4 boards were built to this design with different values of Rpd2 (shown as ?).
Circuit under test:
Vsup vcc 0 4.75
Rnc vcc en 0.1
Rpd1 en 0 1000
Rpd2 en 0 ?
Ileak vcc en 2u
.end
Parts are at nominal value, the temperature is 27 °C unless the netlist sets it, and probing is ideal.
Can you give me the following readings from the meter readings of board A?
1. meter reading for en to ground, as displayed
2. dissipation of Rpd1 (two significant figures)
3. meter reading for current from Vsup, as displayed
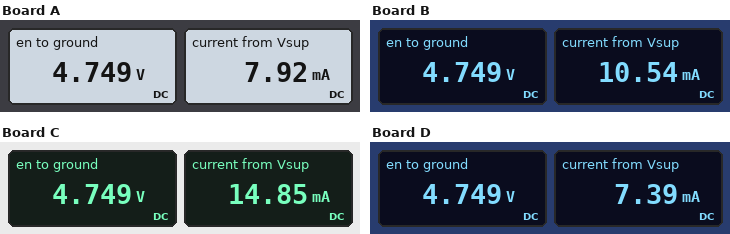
4.749 V
23 mW
7.92 mA
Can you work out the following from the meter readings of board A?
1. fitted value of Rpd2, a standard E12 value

1.5 kΩ
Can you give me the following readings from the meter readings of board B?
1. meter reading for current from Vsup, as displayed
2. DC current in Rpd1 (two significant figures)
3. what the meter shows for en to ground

10.54 mA
4.7 mA
4.749 V
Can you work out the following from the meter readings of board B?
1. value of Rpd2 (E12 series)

820 Ω
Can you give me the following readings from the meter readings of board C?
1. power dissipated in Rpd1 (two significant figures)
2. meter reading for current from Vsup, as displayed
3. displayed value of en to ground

23 mW
14.85 mA
4.749 V
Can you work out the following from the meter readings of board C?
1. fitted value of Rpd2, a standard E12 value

470 Ω
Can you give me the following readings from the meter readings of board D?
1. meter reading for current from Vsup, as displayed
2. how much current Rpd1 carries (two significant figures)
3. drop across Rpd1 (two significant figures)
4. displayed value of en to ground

7.39 mA
4.7 mA
4.7 V
4.749 V
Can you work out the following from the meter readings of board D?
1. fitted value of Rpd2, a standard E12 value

1.8 kΩ
